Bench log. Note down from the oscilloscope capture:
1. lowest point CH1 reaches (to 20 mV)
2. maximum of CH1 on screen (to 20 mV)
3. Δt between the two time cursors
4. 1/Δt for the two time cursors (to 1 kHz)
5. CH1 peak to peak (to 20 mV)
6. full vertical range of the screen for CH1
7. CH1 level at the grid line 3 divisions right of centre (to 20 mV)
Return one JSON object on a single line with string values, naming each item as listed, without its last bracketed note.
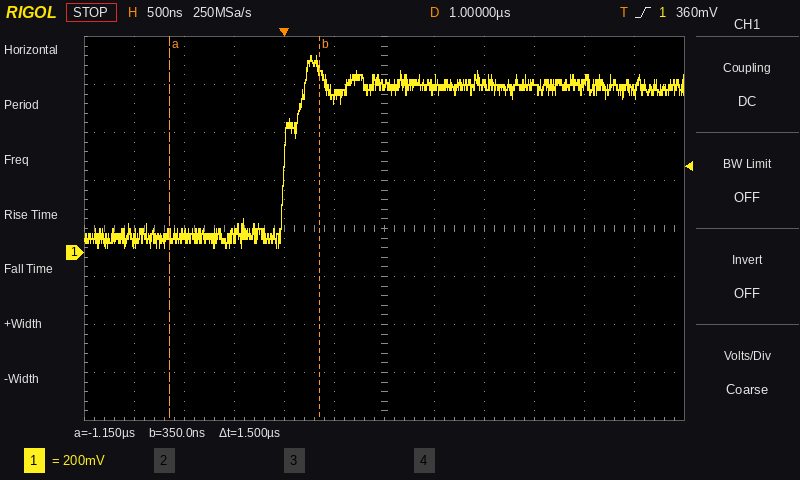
{"lowest point CH1 reaches": "20 mV", "maximum of CH1 on screen": "820 mV", "Δt between the two time cursors": "1.5 µs", "1/Δt for the two time cursors": "667 kHz", "CH1 peak to peak": "800 mV", "full vertical range of the screen for CH1": "1.6 V", "CH1 level at the grid line 3 divisions right of centre": "700 mV"}
